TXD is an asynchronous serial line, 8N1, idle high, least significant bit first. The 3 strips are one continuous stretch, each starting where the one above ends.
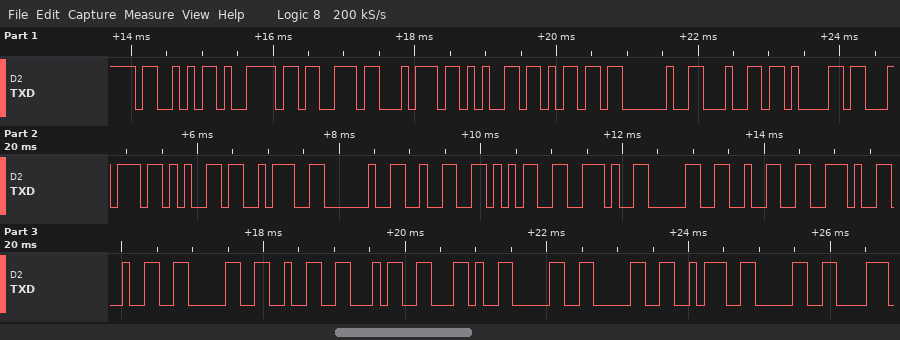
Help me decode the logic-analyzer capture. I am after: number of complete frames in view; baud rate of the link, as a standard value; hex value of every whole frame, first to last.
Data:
28
9600 baud
0x53 0x79 0x73 0x74 0x65 0x6D 0x20 0x64 0x61 0x74 0x65 0x3A 0x20 0x32 0x35 0x2E 0x30 0x32 0x2E 0x32 0x30 0x32 0x34 0x2C 0x30 0x30 0x3A 0x30
